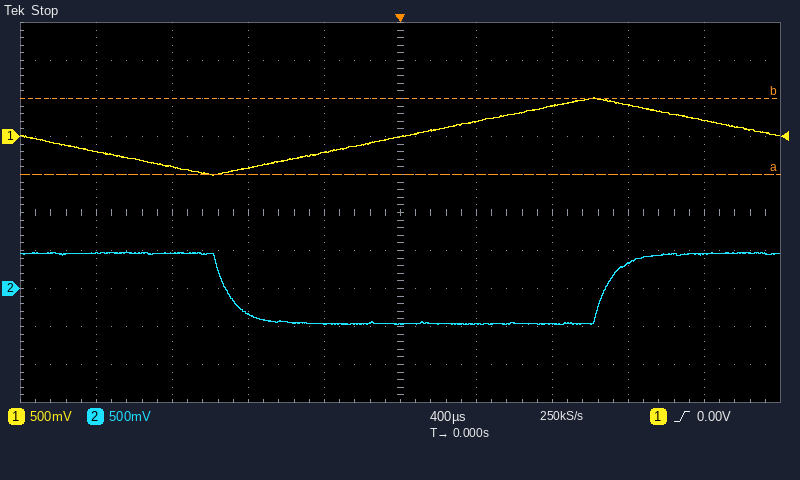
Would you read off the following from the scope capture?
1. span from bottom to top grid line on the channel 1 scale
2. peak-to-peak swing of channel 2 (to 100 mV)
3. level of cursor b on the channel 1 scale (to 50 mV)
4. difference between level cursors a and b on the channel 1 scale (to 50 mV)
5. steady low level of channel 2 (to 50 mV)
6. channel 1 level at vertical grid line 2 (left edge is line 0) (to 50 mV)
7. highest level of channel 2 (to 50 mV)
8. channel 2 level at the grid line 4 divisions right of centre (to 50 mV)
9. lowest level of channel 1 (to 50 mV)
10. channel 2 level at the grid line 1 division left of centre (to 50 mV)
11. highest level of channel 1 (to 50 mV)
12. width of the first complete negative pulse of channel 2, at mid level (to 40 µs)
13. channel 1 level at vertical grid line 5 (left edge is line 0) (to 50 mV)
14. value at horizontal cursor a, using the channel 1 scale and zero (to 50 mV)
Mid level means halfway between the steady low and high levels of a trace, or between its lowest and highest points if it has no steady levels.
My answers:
5 V
1.00 V
500 mV
1.00 V
-450 mV
-400 mV
500 mV
450 mV
-500 mV
-450 mV
500 mV
2.00 ms
0 mV
-500 mV
